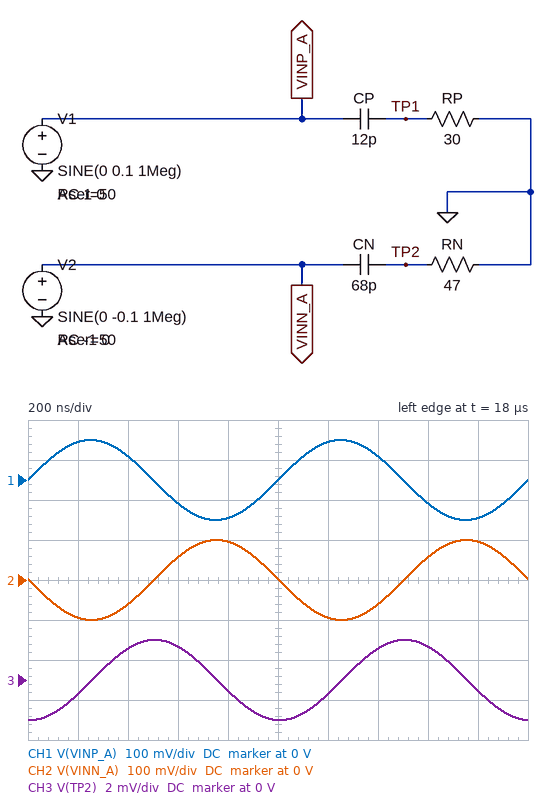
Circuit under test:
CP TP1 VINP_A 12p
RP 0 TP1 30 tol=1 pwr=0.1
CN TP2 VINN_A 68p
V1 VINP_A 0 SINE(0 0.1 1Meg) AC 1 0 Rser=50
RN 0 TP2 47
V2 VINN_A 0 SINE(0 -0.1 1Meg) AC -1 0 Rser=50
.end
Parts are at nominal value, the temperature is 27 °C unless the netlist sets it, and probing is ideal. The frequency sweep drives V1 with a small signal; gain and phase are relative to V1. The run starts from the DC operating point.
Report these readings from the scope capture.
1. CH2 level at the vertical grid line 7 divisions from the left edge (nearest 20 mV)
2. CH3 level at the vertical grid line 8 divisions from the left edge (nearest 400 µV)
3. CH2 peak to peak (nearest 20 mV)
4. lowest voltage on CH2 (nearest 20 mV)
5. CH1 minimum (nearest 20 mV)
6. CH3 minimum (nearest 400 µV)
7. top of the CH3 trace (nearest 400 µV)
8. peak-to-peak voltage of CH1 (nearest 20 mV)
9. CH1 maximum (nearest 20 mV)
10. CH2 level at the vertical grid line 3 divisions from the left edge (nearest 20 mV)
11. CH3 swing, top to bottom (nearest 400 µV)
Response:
-60 mV
1.6 mV
200 mV
-100 mV
-100 mV
-2.0 mV
2.0 mV
200 mV
100 mV
60 mV
4.0 mV
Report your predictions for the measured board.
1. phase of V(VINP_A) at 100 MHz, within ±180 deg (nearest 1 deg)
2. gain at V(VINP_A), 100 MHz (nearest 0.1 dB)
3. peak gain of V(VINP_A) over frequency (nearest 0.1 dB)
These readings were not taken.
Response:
-18 deg
-1.1 dB
0 dB
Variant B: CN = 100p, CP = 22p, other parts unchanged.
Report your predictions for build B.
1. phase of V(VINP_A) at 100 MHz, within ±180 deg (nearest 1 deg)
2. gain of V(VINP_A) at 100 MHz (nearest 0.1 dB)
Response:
-25 deg
-2.8 dB
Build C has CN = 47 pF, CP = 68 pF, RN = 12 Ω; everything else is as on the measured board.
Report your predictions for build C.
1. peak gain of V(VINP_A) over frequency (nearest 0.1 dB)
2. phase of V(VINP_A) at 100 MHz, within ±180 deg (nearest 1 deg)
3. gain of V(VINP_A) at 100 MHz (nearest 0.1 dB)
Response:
0 dB
-22 deg
-6.8 dB
